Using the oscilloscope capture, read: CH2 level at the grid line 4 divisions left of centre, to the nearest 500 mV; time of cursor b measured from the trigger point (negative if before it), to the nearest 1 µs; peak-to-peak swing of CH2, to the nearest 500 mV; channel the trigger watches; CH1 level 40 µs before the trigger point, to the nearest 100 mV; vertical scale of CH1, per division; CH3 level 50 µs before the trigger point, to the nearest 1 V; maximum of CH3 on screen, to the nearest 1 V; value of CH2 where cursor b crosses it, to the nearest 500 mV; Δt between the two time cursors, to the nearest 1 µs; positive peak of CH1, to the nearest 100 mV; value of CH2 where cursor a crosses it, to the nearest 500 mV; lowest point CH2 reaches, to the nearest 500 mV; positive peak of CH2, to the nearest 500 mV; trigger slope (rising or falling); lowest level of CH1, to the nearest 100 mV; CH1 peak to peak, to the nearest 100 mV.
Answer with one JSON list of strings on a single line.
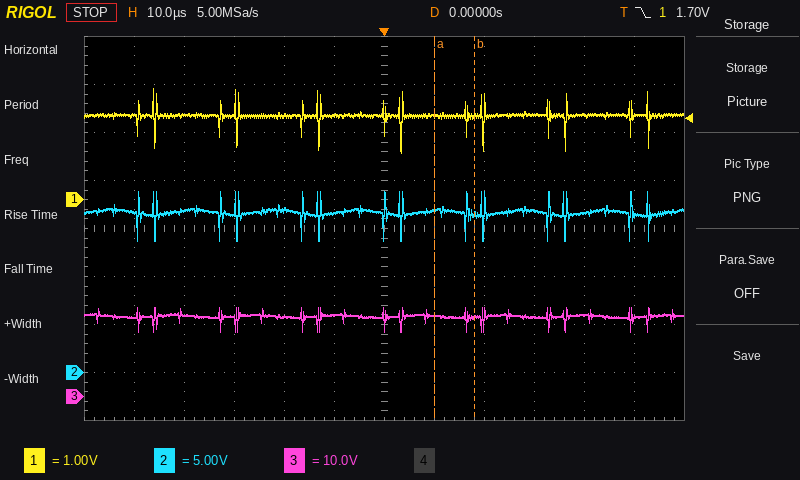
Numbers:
["17.0 V", "+18 µs", "5.0 V", "CH1", "1.8 V", "1 V", "17 V", "19 V", "16.5 V", "8 µs", "2.3 V", "17.0 V", "14.0 V", "19.0 V", "falling", "1.0 V", "1.3 V"]
